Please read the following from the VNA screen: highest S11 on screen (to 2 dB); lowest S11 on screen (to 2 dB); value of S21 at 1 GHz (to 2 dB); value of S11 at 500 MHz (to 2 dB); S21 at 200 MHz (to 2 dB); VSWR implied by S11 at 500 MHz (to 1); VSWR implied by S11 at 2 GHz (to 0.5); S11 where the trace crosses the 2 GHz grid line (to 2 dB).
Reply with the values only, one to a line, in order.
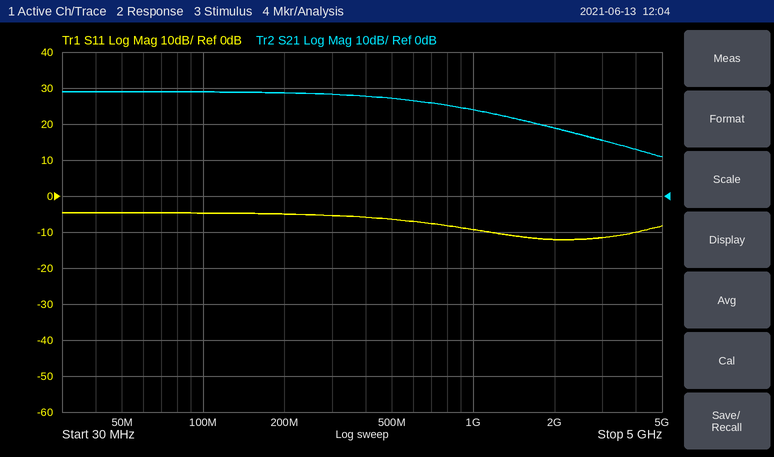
-4 dB
-12 dB
24 dB
-6 dB
28 dB
3
1.5
-12 dB
